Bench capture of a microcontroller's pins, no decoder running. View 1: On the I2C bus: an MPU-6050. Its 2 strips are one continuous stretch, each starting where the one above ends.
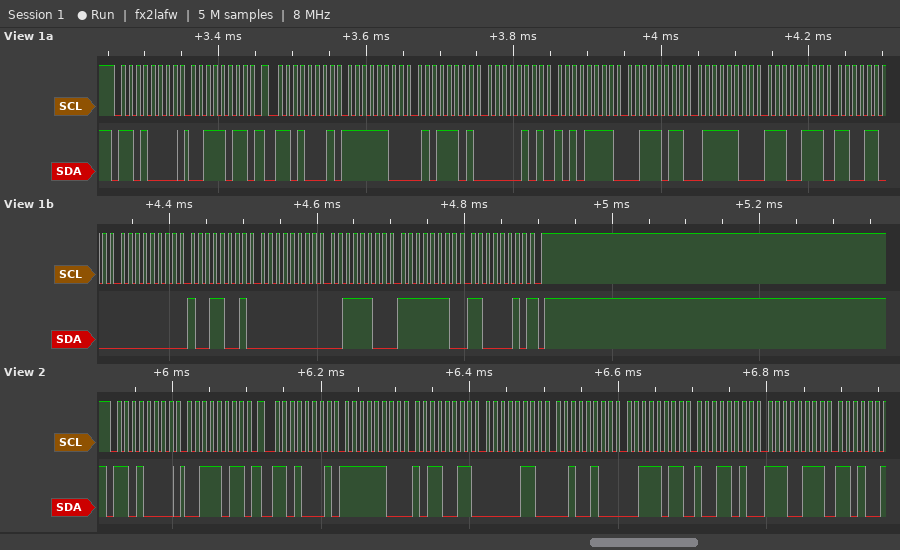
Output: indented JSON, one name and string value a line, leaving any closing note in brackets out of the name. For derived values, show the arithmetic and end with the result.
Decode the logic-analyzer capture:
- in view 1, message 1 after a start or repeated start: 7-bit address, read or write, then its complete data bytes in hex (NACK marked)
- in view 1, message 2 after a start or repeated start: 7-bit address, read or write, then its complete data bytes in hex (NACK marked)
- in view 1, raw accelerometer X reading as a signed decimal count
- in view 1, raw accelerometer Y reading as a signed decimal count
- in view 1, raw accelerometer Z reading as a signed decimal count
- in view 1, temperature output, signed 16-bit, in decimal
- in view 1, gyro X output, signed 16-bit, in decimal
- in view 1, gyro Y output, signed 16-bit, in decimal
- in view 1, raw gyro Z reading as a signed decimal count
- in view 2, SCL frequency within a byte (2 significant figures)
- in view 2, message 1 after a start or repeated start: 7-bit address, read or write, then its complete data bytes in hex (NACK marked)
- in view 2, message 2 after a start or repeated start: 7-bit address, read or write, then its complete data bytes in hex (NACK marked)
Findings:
{
  "in view 1, message 1 after a start or repeated start: 7-bit address, read or write, then its complete data bytes in hex": "0x68 write: 3B",
  "in view 1, message 2 after a start or repeated start: 7-bit address, read or write, then its complete data bytes in hex": "0x68 read: FC 5D 05 AF 3B 7C E7 CC 00 99 00 3C FE C2 NACK",
  "in view 1, raw accelerometer X reading as a signed decimal count": "0xFC5D = -931",
  "in view 1, raw accelerometer Y reading as a signed decimal count": "0x05AF = 1455",
  "in view 1, raw accelerometer Z reading as a signed decimal count": "0x3B7C = 15228",
  "in view 1, temperature output, signed 16-bit, in decimal": "0xE7CC = -6196",
  "in view 1, gyro X output, signed 16-bit, in decimal": "0x0099 = 153",
  "in view 1, gyro Y output, signed 16-bit, in decimal": "0x003C = 60",
  "in view 1, raw gyro Z reading as a signed decimal count": "0xFEC2 = -318",
  "in view 2, SCL frequency within a byte": "100 kHz",
  "in view 2, message 1 after a start or repeated start: 7-bit address, read or write, then its complete data bytes in hex": "0x68 write: 3B",
  "in view 2, message 2 after a start or repeated start: 7-bit address, read or write, then its complete data bytes in hex": "0x68 read: FC B3 06 24 3B 9A E7"
}
